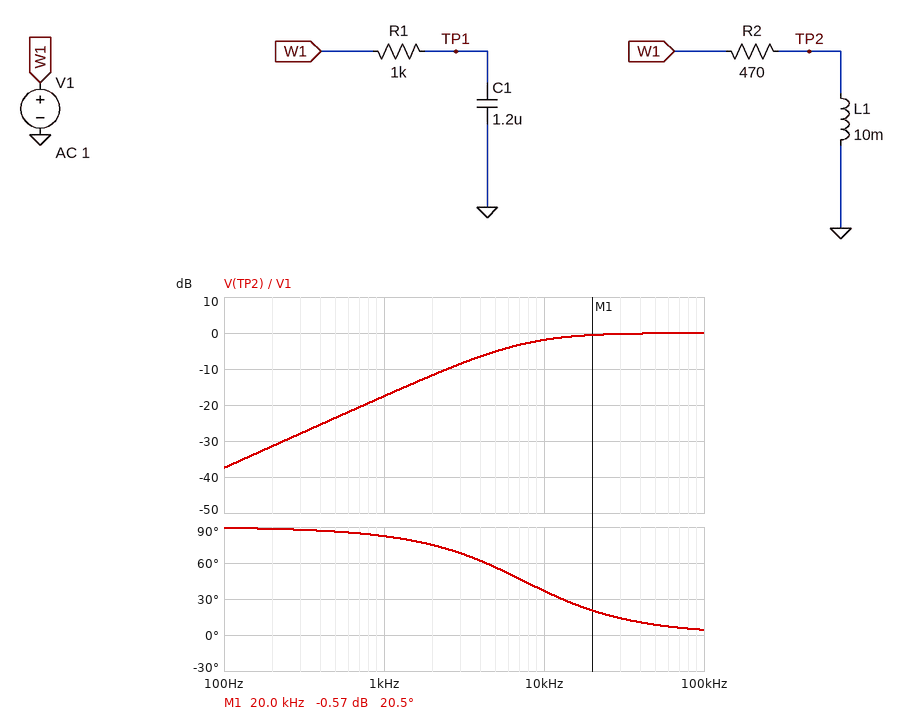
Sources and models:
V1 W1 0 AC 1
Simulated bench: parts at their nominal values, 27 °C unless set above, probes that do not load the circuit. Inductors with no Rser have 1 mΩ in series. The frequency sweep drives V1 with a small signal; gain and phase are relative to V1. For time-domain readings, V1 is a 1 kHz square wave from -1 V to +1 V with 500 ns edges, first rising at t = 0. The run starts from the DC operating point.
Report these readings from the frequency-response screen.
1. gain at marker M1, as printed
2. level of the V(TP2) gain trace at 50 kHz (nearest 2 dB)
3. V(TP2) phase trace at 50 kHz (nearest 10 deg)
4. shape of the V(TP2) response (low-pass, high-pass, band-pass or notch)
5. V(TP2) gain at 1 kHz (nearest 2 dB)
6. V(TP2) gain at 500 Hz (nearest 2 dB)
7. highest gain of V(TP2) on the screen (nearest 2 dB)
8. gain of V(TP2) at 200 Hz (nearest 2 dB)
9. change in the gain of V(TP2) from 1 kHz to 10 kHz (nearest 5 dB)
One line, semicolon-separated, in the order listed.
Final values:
-0.57 dB; 0 dB; 10 deg; high-pass; -18 dB; -24 dB; 0 dB; -32 dB; 15 dB
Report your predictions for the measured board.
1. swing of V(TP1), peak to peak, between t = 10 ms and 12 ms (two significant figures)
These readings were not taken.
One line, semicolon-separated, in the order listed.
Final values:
410 mV
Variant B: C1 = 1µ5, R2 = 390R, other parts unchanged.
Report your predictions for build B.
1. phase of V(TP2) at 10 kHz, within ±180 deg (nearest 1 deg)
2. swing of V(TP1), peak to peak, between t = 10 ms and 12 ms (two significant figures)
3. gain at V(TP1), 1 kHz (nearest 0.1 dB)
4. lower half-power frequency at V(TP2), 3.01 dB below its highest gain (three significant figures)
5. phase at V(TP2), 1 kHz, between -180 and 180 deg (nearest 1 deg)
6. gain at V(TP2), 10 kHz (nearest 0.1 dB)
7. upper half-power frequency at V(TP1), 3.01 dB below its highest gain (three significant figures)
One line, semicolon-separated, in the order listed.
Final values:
32 deg; 330 mV; -19.5 dB; 6.21 kHz; 81 deg; -1.4 dB; 106 Hz
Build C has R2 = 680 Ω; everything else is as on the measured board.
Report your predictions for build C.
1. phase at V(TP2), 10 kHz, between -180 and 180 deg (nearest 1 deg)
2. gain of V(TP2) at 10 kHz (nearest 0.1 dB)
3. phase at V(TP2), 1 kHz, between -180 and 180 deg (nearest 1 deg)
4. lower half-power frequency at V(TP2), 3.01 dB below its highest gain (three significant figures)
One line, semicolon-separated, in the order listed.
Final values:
47 deg; -3.4 dB; 85 deg; 10.8 kHz
